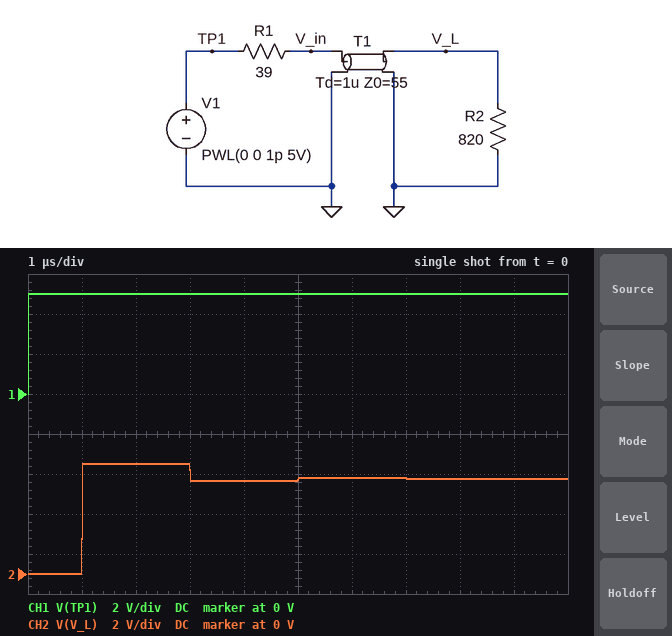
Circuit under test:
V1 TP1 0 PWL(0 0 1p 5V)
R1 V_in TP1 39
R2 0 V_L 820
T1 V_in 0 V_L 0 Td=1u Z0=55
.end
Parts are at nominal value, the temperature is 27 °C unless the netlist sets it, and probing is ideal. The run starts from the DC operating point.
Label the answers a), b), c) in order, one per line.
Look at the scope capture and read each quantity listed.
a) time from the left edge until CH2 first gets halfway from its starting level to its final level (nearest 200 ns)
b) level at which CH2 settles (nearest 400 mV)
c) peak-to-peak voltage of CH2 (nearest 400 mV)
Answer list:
a) 1.0 µs
b) 4.8 V
c) 5.6 V
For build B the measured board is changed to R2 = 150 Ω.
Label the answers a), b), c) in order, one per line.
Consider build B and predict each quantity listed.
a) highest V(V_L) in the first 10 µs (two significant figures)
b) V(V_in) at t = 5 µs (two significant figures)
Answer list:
a) 4.3 V
b) 4.0 V
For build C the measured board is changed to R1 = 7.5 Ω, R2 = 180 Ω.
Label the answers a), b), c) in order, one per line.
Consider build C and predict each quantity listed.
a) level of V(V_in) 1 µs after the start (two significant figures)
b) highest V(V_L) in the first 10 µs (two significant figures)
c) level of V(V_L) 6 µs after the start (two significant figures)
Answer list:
a) 4.4 V
b) 6.7 V
c) 5.1 V
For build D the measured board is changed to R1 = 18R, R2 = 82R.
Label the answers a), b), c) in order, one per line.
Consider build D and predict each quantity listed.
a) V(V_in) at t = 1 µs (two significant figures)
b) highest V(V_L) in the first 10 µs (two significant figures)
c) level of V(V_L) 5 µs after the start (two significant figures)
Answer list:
a) 3.8 V
b) 4.5 V
c) 4.1 V
